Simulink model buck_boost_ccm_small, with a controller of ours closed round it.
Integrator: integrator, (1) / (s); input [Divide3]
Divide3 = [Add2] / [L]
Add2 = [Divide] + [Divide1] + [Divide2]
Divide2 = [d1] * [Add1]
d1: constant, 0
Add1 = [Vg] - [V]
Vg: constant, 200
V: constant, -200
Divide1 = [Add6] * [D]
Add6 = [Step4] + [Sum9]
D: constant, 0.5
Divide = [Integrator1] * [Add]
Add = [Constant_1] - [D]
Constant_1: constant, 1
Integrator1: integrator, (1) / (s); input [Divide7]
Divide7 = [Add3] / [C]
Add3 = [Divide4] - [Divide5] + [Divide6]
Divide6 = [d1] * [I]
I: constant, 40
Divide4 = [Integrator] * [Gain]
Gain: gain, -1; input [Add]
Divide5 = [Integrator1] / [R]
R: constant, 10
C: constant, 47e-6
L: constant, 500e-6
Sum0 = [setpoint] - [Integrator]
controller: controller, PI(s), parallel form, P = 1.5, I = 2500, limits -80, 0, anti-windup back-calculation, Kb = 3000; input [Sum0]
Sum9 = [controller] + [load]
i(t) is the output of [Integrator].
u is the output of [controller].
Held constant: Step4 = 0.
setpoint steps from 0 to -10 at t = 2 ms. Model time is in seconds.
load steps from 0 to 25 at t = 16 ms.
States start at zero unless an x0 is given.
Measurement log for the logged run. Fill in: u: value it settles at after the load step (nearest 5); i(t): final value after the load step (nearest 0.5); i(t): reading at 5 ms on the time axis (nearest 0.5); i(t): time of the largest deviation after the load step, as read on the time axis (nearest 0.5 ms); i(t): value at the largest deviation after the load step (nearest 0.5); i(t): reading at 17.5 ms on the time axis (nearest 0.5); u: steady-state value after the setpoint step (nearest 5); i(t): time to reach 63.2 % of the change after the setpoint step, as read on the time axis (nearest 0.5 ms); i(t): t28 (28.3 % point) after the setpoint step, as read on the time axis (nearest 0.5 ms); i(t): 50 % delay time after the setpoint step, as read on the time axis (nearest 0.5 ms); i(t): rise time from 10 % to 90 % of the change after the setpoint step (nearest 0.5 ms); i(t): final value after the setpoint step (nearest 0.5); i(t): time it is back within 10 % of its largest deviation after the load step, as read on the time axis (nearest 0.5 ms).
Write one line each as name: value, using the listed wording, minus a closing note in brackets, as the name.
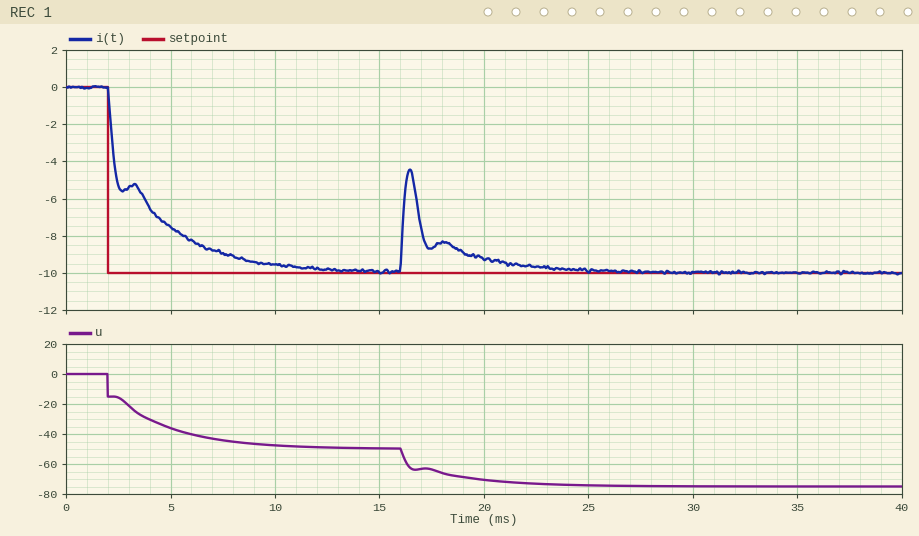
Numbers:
u: value it settles at after the load step: -75
i(t): final value after the load step: -10.0
i(t): reading at 5 ms on the time axis: -7.5
i(t): time of the largest deviation after the load step, as read on the time axis: 16.5 ms
i(t): value at the largest deviation after the load step: -4.5
i(t): reading at 17.5 ms on the time axis: -8.5
u: steady-state value after the setpoint step: -50
i(t): time to reach 63.2 % of the change after the setpoint step, as read on the time axis: 4.0 ms
i(t): t28 (28.3 % point) after the setpoint step, as read on the time axis: 2.0 ms
i(t): 50 % delay time after the setpoint step, as read on the time axis: 2.5 ms
i(t): rise time from 10 % to 90 % of the change after the setpoint step: 5.5 ms
i(t): final value after the setpoint step: -10.0
i(t): time it is back within 10 % of its largest deviation after the load step, as read on the time axis: 21.0 ms
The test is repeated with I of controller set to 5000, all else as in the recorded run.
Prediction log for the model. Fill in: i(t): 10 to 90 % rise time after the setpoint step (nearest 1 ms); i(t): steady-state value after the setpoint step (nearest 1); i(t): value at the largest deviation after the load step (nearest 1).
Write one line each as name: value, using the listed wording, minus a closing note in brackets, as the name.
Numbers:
i(t): 10 to 90 % rise time after the setpoint step: 3 ms
i(t): steady-state value after the setpoint step: -10
i(t): value at the largest deviation after the load step: -5
